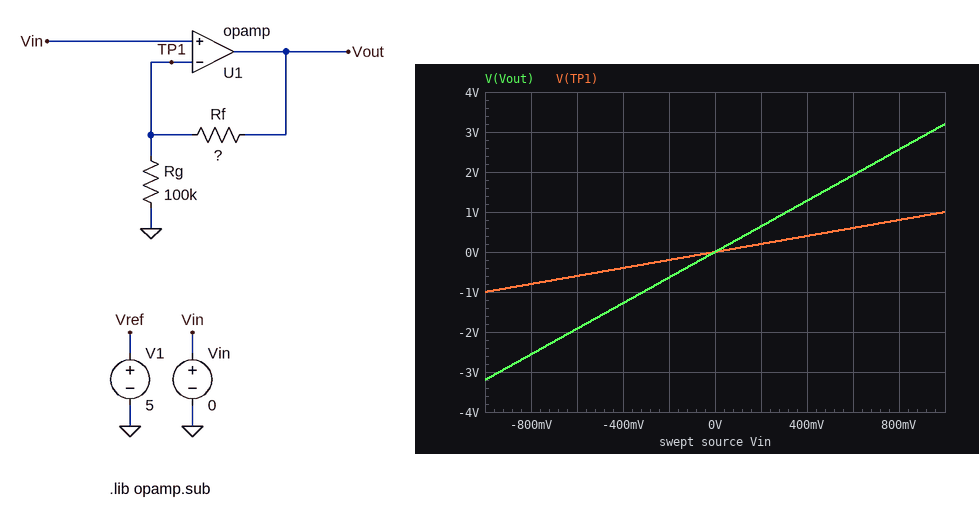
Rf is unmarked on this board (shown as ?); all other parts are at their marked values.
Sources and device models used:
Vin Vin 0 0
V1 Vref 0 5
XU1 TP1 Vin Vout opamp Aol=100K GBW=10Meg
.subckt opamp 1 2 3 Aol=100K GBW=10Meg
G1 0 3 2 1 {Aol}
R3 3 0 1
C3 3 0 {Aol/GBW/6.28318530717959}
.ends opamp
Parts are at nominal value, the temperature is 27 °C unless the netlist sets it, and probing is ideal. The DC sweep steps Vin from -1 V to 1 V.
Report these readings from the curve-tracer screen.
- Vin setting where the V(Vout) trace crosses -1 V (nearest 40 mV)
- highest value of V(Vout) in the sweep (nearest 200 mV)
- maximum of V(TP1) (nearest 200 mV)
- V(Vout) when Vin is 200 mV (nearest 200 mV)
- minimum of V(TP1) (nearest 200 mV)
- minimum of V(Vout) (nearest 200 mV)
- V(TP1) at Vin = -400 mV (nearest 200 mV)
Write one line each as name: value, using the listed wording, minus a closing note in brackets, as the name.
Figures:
Vin setting where the V(Vout) trace crosses -1 V: -320 mV
highest value of V(Vout) in the sweep: 3.2 V
maximum of V(TP1): 1.0 V
V(Vout) when Vin is 200 mV: 600 mV
minimum of V(TP1): -1.0 V
minimum of V(Vout): -3.2 V
V(TP1) at Vin = -400 mV: -400 mV
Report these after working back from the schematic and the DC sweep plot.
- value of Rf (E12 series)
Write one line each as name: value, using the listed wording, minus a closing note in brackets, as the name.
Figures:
value of Rf: 220 kΩ
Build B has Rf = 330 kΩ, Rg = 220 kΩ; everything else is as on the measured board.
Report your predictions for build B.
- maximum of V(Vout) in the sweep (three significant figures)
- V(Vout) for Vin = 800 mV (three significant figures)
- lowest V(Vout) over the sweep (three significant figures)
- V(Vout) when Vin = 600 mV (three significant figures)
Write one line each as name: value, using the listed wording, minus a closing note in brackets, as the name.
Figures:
maximum of V(Vout) in the sweep: 2.50 V
V(Vout) for Vin = 800 mV: 2.00 V
lowest V(Vout) over the sweep: -2.50 V
V(Vout) when Vin = 600 mV: 1.50 V
